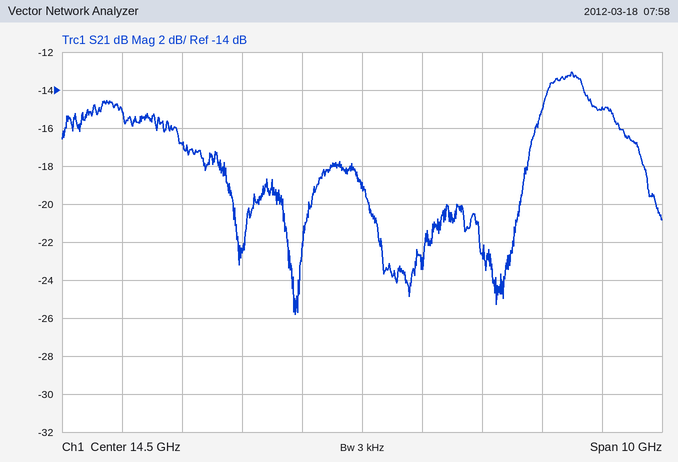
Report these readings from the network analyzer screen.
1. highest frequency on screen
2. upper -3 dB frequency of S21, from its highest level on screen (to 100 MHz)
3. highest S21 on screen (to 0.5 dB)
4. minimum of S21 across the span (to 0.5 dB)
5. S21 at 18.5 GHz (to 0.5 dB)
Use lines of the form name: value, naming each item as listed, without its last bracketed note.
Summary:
highest frequency on screen: 19.5 GHz
upper -3 dB frequency of S21, from its highest level on screen: 18.8 GHz
highest S21 on screen: -13.0 dB
minimum of S21 across the span: -26.0 dB
S21 at 18.5 GHz: -15.0 dB
